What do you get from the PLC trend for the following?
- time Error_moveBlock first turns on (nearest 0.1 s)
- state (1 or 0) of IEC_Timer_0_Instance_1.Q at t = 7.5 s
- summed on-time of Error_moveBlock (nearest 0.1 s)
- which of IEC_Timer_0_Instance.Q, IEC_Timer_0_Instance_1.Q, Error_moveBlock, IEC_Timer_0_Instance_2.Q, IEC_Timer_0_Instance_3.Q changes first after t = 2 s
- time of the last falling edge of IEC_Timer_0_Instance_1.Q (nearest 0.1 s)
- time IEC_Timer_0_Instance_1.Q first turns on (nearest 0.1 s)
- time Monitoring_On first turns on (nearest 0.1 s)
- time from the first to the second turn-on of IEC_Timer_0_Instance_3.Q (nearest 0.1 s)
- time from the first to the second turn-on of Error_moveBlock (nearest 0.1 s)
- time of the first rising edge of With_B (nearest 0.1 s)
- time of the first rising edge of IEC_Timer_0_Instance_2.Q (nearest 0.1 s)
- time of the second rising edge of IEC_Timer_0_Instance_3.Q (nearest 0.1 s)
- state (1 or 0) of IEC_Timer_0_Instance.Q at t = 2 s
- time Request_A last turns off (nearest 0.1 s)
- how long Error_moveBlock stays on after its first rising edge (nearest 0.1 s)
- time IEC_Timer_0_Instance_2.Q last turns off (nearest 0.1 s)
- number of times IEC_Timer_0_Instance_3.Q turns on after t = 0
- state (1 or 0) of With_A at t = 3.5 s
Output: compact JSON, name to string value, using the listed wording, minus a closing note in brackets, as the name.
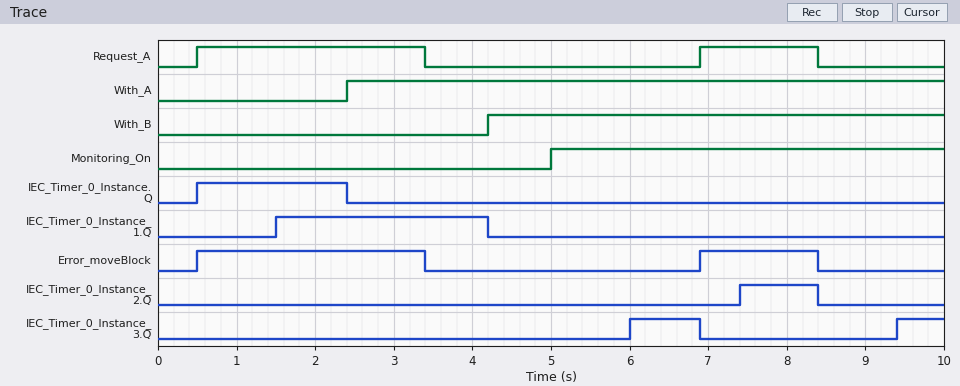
{"time Error_moveBlock first turns on": "0.5 s", "state (1 or 0) of IEC_Timer_0_Instance_1.Q at t = 7.5 s": "0", "summed on-time of Error_moveBlock": "4.4 s", "which of IEC_Timer_0_Instance.Q, IEC_Timer_0_Instance_1.Q, Error_moveBlock, IEC_Timer_0_Instance_2.Q, IEC_Timer_0_Instance_3.Q changes first after t = 2 s": "IEC_Timer_0_Instance.Q", "time of the last falling edge of IEC_Timer_0_Instance_1.Q": "4.2 s", "time IEC_Timer_0_Instance_1.Q first turns on": "1.5 s", "time Monitoring_On first turns on": "5.0 s", "time from the first to the second turn-on of IEC_Timer_0_Instance_3.Q": "3.4 s", "time from the first to the second turn-on of Error_moveBlock": "6.4 s", "time of the first rising edge of With_B": "4.2 s", "time of the first rising edge of IEC_Timer_0_Instance_2.Q": "7.4 s", "time of the second rising edge of IEC_Timer_0_Instance_3.Q": "9.4 s", "state (1 or 0) of IEC_Timer_0_Instance.Q at t = 2 s": "1", "time Request_A last turns off": "8.4 s", "how long Error_moveBlock stays on after its first rising edge": "2.9 s", "time IEC_Timer_0_Instance_2.Q last turns off": "8.4 s", "number of times IEC_Timer_0_Instance_3.Q turns on after t = 0": "2", "state (1 or 0) of With_A at t = 3.5 s": "1"}
